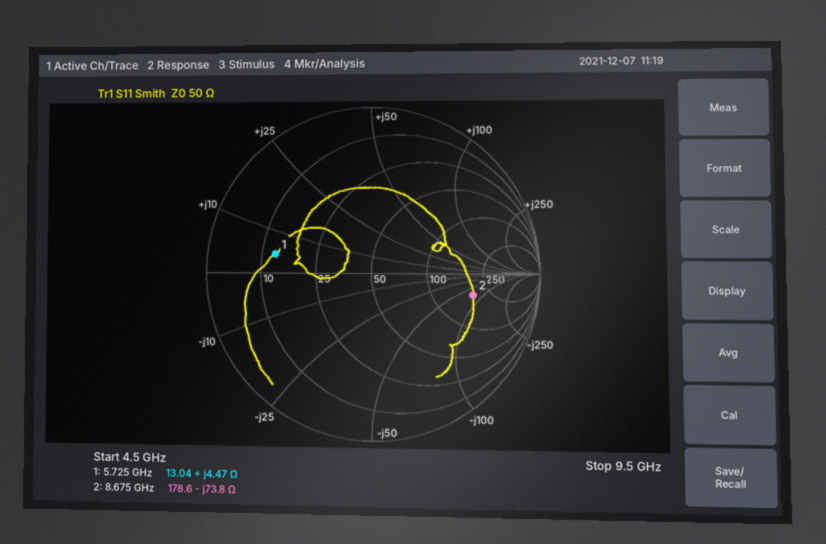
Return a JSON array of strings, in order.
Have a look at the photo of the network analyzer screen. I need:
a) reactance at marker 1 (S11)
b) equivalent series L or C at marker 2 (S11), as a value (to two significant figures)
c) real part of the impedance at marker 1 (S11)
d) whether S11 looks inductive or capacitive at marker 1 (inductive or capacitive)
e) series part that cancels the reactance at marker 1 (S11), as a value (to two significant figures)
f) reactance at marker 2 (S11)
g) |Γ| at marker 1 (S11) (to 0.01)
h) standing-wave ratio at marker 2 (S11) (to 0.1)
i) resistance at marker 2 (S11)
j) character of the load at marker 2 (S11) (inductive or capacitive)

["+4.47 Ω", "250 fF", "13.04 Ω", "inductive", "6.2 pF", "-73.8 Ω", "0.59", "4.2", "178.6 Ω", "capacitive"]
